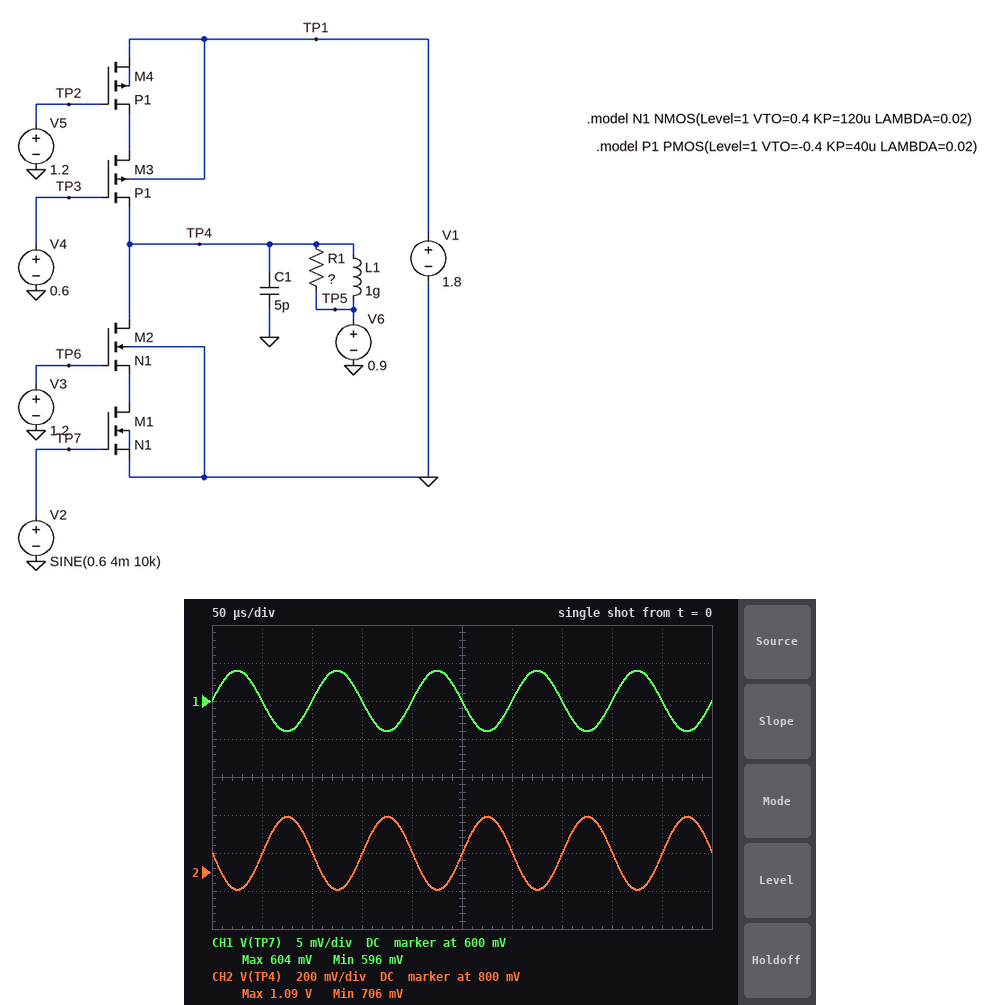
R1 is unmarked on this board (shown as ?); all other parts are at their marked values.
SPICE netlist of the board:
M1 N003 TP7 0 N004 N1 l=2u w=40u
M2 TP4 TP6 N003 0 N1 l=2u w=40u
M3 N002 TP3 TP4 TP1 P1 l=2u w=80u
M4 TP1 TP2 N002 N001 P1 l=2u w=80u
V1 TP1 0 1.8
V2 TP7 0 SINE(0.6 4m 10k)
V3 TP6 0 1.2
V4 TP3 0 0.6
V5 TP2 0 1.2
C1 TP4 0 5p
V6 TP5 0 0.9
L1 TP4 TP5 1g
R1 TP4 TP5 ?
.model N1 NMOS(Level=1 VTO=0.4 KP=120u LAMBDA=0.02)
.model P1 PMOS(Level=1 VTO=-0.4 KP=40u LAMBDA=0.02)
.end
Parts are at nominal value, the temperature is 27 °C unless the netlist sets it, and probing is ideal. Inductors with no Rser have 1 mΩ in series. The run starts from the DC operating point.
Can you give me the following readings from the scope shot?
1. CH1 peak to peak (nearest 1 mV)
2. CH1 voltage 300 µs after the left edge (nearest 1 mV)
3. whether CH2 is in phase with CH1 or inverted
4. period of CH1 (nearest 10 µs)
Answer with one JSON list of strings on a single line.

["8 mV", "600 mV", "inverted", "100 µs"]
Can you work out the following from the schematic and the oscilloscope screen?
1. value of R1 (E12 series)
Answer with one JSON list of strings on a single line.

["100 kΩ"]
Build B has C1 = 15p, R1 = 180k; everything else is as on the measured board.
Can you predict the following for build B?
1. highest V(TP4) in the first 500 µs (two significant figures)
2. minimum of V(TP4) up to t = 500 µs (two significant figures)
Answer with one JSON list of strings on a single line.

["1.2 V", "570 mV"]
